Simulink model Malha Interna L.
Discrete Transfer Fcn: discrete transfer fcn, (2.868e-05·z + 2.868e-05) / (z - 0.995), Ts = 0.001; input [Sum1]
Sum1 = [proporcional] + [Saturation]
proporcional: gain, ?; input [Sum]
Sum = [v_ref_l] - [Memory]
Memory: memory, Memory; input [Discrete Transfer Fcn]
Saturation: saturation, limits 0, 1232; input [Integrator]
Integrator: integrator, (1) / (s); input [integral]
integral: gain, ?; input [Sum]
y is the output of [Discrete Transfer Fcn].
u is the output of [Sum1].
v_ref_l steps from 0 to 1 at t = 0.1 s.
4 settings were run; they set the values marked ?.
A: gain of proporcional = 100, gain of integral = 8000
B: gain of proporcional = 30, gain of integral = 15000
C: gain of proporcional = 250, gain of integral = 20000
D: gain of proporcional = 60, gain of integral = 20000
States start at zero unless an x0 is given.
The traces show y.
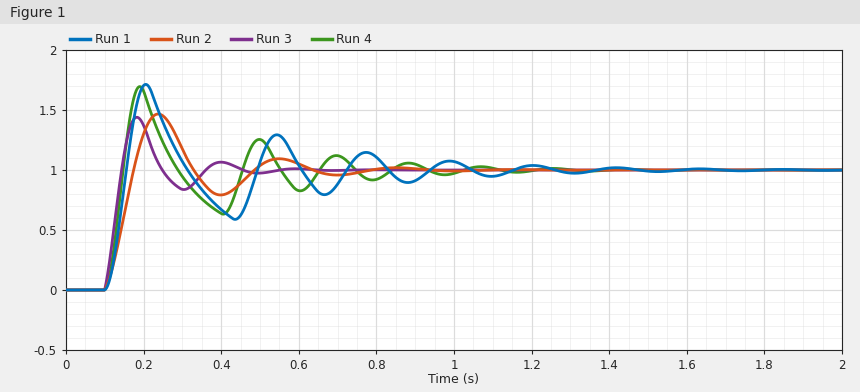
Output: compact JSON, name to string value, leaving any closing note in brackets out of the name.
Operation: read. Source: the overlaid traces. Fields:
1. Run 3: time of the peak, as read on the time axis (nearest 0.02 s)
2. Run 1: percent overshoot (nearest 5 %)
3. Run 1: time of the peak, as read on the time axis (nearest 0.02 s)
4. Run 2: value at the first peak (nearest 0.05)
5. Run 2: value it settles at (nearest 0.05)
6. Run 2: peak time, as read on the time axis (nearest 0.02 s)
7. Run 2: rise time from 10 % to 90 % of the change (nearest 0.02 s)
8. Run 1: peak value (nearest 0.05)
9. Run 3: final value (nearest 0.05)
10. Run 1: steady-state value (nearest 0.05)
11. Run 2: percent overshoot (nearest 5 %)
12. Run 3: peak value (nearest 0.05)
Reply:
{"Run 3: time of the peak, as read on the time axis": "0.18 s", "Run 1: percent overshoot": "70 %", "Run 1: time of the peak, as read on the time axis": "0.20 s", "Run 2: value at the first peak": "1.45", "Run 2: value it settles at": "1.00", "Run 2: peak time, as read on the time axis": "0.24 s", "Run 2: rise time from 10 % to 90 % of the change": "0.06 s", "Run 1: peak value": "1.70", "Run 3: final value": "1.00", "Run 1: steady-state value": "1.00", "Run 2: percent overshoot": "45 %", "Run 3: peak value": "1.45"}
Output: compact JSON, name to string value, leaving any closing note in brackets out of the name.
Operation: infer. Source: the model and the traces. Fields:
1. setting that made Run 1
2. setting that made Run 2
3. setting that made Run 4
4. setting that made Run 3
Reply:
{"setting that made Run 1": "B", "setting that made Run 2": "A", "setting that made Run 4": "D", "setting that made Run 3": "C"}
